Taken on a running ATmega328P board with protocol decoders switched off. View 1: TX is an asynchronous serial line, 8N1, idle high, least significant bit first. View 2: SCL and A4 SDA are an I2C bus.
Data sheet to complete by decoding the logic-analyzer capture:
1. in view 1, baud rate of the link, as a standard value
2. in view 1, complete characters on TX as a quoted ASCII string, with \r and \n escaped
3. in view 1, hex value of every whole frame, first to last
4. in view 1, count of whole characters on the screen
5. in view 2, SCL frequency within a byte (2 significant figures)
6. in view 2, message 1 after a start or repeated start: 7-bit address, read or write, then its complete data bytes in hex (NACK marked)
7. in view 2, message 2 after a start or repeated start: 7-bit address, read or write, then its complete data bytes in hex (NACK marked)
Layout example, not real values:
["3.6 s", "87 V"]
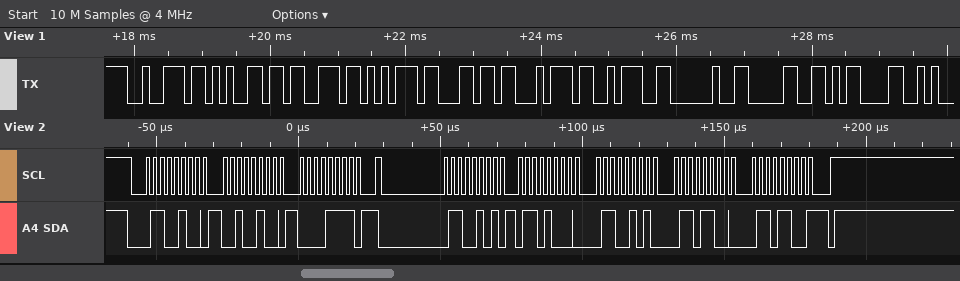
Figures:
["9600 baud", "\"result: 0\\r\"", "0x72 0x65 0x73 0x75 0x6C 0x74 0x3A 0x20 0x30 0x0D", "10", "400 kHz", "0x32 write: 24 0F", "0x32 read: 68 65 6C 6C NACK"]
